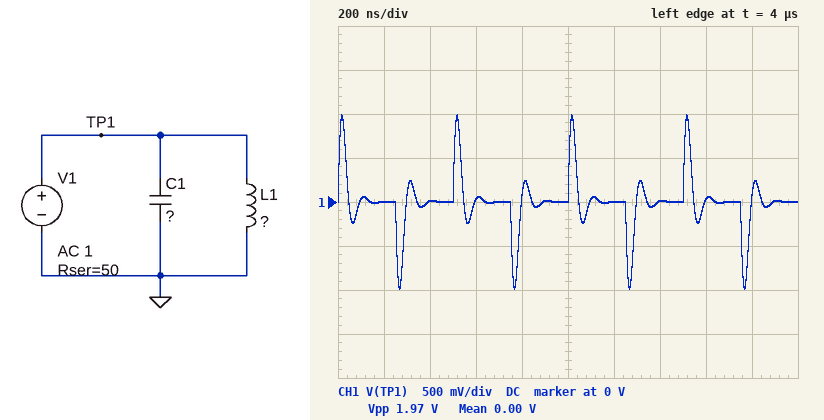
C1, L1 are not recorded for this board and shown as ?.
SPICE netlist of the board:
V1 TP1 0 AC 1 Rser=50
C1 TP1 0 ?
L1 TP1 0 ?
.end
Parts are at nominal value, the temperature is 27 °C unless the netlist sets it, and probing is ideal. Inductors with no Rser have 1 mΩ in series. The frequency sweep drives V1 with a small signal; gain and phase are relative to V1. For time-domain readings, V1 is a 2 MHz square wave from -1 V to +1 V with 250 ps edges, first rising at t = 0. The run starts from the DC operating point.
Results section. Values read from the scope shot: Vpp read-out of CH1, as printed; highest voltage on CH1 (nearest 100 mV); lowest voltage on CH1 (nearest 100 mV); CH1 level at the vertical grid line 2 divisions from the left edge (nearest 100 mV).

1.97 V
1.0 V
-1.0 V
0 V
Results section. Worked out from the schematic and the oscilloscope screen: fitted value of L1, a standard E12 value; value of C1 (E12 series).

560 nH
330 pF
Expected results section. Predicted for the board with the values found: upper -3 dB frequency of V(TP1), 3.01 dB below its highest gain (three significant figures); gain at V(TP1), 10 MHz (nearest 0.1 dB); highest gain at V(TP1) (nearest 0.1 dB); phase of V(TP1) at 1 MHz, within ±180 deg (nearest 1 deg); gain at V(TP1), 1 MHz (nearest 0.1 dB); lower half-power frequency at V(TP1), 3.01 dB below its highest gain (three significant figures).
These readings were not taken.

17.5 MHz
-0.6 dB
0 dB
86 deg
-23.0 dB
7.84 MHz
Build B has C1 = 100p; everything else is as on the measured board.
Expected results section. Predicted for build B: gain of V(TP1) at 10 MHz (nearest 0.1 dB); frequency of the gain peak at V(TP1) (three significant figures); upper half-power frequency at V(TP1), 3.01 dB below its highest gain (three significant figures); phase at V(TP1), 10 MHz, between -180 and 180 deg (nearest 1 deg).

-3.5 dB
21.3 MHz
42.5 MHz
48 deg
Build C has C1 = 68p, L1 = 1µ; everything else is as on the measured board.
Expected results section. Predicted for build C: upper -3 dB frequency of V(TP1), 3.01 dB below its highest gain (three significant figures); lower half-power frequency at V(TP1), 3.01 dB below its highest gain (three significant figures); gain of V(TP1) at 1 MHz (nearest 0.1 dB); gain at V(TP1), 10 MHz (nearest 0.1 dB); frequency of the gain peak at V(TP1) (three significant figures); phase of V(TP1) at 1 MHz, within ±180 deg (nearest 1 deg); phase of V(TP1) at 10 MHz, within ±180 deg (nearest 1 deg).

53.7 MHz
6.93 MHz
-18.1 dB
-1.3 dB
19.3 MHz
83 deg
30 deg
